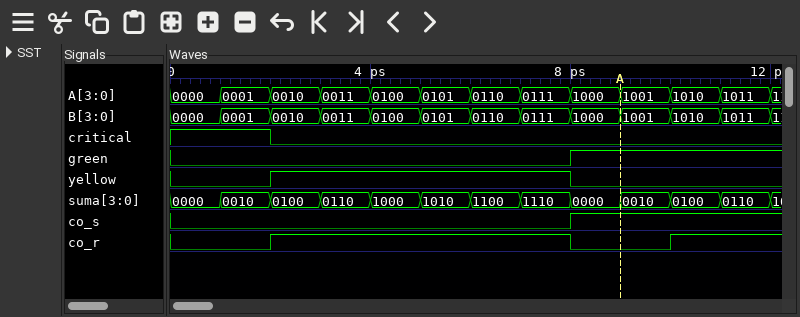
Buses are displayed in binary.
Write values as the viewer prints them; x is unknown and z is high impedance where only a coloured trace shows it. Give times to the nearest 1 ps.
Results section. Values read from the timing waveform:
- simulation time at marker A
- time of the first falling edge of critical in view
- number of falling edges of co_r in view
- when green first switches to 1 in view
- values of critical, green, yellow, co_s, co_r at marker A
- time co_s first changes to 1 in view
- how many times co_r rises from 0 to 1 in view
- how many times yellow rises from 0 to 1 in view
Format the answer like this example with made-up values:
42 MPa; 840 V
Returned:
9 ps; 2 ps; 1; 8 ps; critical=0, green=1, yellow=0, co_s=1, co_r=0; 8 ps; 2; 1
